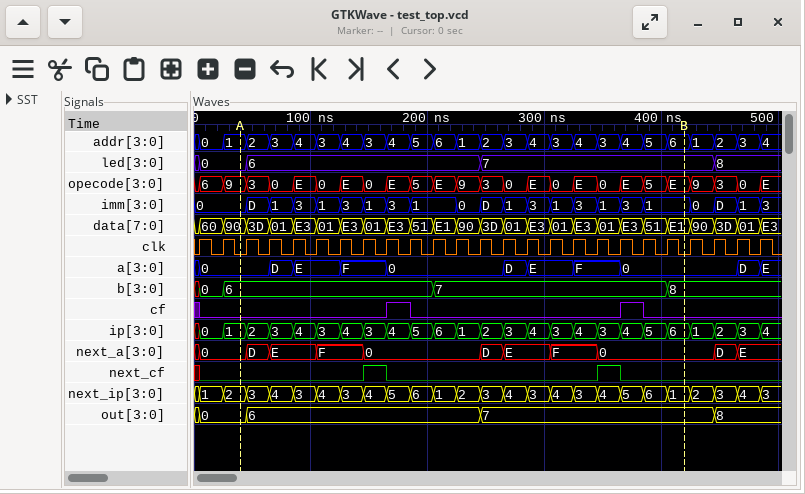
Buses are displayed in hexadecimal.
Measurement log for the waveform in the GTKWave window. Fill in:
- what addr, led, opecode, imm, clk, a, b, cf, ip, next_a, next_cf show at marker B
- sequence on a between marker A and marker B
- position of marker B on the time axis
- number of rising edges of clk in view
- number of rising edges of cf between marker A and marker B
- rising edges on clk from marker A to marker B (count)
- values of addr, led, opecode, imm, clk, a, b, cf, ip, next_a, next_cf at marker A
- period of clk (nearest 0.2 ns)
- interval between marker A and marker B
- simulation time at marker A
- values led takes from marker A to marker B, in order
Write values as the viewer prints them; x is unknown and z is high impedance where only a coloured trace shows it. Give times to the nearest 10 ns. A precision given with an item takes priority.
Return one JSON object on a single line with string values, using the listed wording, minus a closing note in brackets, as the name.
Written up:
{"what addr, led, opecode, imm, clk, a, b, cf, ip, next_a, next_cf show at marker B": "addr=6, led=7, opecode=E, imm=1, clk=0, a=0, b=8, cf=0, ip=6, next_a=0, next_cf=0", "sequence on a between marker A and marker B": "0, D, E, F, 0, D, E, F, 0", "position of marker B on the time axis": "420 ns", "number of rising edges of clk in view": "25", "number of rising edges of cf between marker A and marker B": "2", "rising edges on clk from marker A to marker B": "19", "values of addr, led, opecode, imm, clk, a, b, cf, ip, next_a, next_cf at marker A": "addr=1, led=0, opecode=9, imm=0, clk=0, a=0, b=6, cf=0, ip=1, next_a=0, next_cf=0", "period of clk": "20 ns", "interval between marker A and marker B": "380 ns", "simulation time at marker A": "40 ns", "values led takes from marker A to marker B, in order": "0, 6, 7"}
